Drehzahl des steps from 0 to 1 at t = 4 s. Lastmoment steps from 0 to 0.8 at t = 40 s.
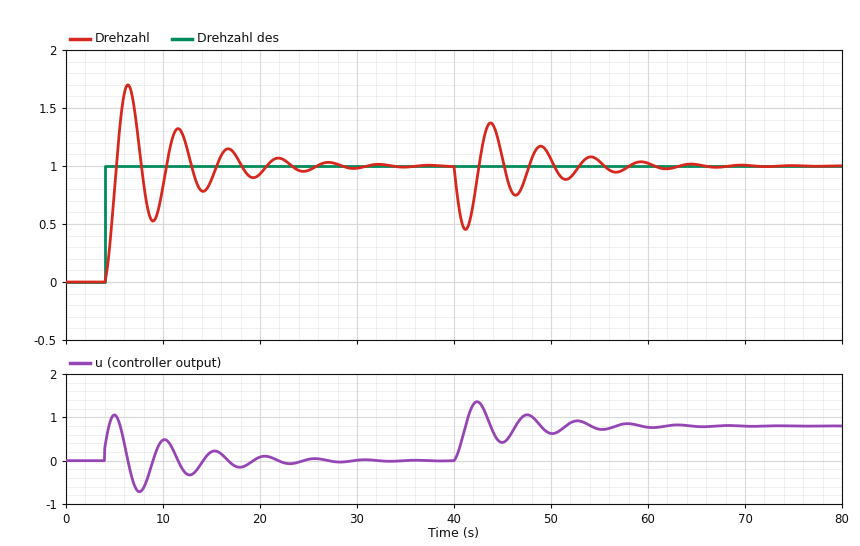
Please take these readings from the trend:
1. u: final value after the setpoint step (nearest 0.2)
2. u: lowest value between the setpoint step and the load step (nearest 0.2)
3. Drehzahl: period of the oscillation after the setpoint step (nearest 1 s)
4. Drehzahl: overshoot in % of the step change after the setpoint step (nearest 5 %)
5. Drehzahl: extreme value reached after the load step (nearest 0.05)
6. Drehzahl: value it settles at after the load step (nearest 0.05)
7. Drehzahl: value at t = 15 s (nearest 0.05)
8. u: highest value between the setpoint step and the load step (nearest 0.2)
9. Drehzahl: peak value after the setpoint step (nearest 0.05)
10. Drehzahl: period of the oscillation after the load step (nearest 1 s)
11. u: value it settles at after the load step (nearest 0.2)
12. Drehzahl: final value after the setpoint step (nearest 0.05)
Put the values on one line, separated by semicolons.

0.0; -0.8; 5 s; 70 %; 0.45; 1.00; 0.90; 1.0; 1.70; 5 s; 0.8; 1.00
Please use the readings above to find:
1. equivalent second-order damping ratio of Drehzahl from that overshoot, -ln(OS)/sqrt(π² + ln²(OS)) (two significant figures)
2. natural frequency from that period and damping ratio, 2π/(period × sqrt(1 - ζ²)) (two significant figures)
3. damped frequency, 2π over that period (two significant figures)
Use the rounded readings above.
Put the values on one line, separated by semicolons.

0.11; 1.3 rad/s; 1.3 rad/s
